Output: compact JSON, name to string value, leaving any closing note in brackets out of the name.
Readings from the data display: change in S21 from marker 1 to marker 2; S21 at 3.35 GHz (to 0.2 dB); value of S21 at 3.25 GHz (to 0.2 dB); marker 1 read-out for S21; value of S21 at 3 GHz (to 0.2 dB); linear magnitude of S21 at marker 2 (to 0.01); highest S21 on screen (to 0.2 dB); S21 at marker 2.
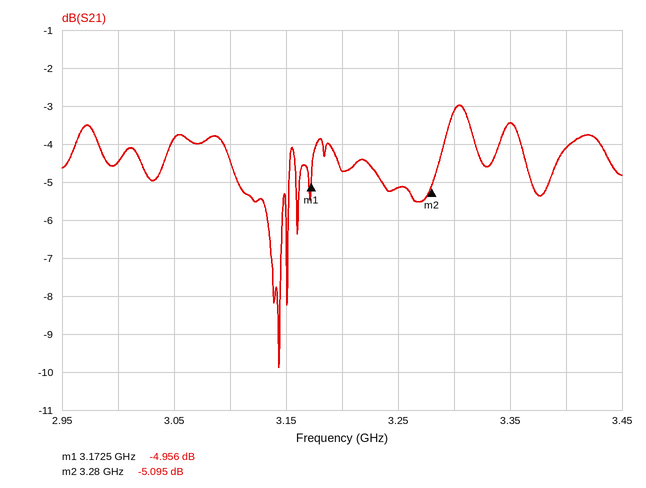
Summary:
{"change in S21 from marker 1 to marker 2": "-0.139 dB", "S21 at 3.35 GHz": "-3.4 dB", "value of S21 at 3.25 GHz": "-5.2 dB", "marker 1 read-out for S21": "-4.956 dB", "value of S21 at 3 GHz": "-4.4 dB", "linear magnitude of S21 at marker 2": "0.56", "highest S21 on screen": "-3.0 dB", "S21 at marker 2": "-5.095 dB"}
